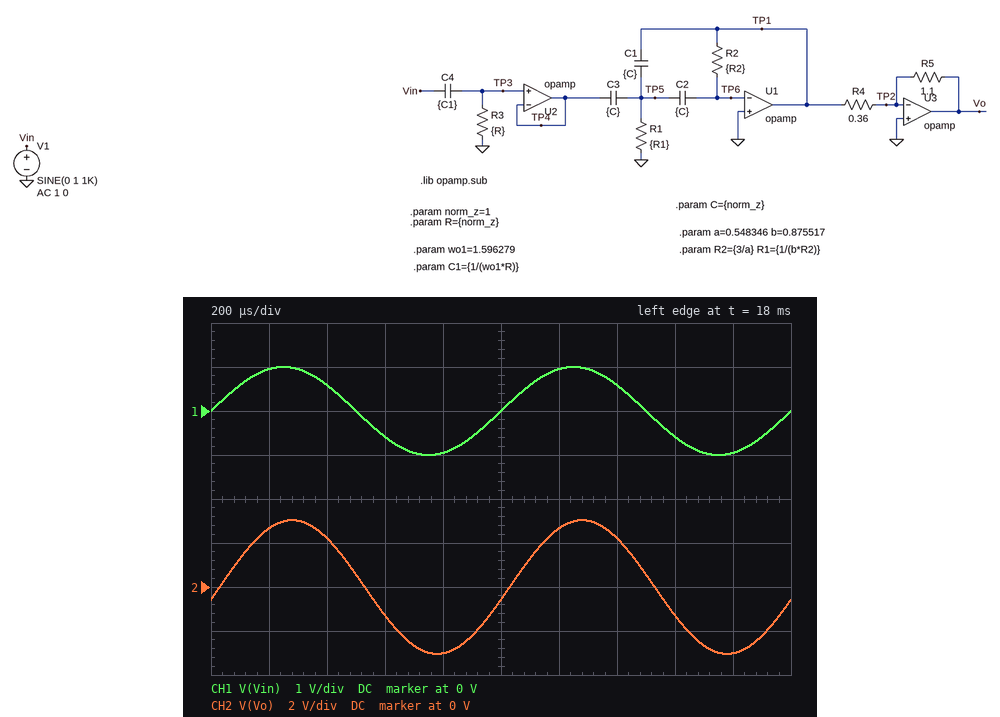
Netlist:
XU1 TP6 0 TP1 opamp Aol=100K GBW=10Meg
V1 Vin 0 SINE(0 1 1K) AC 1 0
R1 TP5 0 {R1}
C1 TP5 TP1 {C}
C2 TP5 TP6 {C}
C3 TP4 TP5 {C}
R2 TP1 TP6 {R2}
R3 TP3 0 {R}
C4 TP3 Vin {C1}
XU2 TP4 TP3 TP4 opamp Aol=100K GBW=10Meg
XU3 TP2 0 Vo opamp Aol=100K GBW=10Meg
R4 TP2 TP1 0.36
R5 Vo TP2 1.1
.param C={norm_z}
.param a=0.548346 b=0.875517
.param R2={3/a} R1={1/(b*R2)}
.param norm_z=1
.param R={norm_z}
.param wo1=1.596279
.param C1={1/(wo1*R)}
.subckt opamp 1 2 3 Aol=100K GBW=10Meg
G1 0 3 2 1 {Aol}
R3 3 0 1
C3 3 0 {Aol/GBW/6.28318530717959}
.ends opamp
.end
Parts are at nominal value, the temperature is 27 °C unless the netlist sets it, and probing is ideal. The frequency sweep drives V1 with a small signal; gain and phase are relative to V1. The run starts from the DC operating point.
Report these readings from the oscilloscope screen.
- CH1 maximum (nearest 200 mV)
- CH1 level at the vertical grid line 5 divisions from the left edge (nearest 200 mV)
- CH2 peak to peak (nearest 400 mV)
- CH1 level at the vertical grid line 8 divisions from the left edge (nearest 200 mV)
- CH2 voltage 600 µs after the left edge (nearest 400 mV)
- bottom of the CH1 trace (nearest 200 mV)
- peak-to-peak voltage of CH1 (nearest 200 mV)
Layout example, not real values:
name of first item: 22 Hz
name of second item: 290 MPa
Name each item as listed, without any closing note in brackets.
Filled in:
CH1 maximum: 1.0 V
CH1 level at the vertical grid line 5 divisions from the left edge: 0 V
CH2 peak to peak: 6.0 V
CH1 level at the vertical grid line 8 divisions from the left edge: -600 mV
CH2 voltage 600 µs after the left edge: -1.2 V
bottom of the CH1 trace: -1.0 V
peak-to-peak voltage of CH1: 2.0 V
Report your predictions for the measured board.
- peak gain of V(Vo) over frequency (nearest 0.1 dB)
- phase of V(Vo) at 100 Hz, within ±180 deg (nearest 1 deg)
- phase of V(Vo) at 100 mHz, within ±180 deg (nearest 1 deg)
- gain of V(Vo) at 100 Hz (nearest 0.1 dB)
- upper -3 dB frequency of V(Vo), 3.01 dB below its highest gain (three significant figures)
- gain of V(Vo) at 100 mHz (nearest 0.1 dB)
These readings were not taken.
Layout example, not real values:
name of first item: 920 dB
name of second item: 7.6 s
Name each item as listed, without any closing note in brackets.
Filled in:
peak gain of V(Vo) over frequency: 9.7 dB
phase of V(Vo) at 100 Hz, within ±180 deg: -1 deg
phase of V(Vo) at 100 mHz, within ±180 deg: -147 deg
gain of V(Vo) at 100 Hz: 9.7 dB
upper -3 dB frequency of V(Vo), 3.01 dB below its highest gain: 11.2 kHz
gain of V(Vo) at 100 mHz: -2.5 dB
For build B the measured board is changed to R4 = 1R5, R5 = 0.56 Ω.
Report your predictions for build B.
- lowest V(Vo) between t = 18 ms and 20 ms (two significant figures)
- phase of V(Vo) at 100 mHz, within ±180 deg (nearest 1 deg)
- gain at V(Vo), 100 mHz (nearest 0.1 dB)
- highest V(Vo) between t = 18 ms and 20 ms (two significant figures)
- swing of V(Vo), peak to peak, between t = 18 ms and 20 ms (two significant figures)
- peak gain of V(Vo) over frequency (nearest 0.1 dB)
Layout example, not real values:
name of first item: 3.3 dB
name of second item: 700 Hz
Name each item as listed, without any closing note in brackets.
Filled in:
lowest V(Vo) between t = 18 ms and 20 ms: -370 mV
phase of V(Vo) at 100 mHz, within ±180 deg: -147 deg
gain at V(Vo), 100 mHz: -20.8 dB
highest V(Vo) between t = 18 ms and 20 ms: 370 mV
swing of V(Vo), peak to peak, between t = 18 ms and 20 ms: 740 mV
peak gain of V(Vo) over frequency: -8.6 dB
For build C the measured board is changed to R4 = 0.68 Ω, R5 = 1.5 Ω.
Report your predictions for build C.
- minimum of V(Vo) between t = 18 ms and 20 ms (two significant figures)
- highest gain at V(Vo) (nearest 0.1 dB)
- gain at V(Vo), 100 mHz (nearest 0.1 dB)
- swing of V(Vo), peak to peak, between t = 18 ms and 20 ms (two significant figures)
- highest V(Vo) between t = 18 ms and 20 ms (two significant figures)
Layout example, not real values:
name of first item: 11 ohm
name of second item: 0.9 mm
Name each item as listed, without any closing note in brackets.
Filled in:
minimum of V(Vo) between t = 18 ms and 20 ms: -2.2 V
highest gain at V(Vo): 6.9 dB
gain at V(Vo), 100 mHz: -5.4 dB
swing of V(Vo), peak to peak, between t = 18 ms and 20 ms: 4.4 V
highest V(Vo) between t = 18 ms and 20 ms: 2.2 V
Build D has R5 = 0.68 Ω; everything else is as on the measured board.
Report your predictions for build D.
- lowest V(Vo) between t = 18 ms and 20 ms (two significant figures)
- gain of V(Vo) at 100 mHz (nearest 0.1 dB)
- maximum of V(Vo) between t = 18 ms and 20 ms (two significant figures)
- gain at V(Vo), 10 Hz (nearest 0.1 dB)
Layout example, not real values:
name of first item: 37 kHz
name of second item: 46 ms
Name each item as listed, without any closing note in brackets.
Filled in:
lowest V(Vo) between t = 18 ms and 20 ms: -1.9 V
gain of V(Vo) at 100 mHz: -6.7 dB
maximum of V(Vo) between t = 18 ms and 20 ms: 1.9 V
gain at V(Vo), 10 Hz: 5.5 dB
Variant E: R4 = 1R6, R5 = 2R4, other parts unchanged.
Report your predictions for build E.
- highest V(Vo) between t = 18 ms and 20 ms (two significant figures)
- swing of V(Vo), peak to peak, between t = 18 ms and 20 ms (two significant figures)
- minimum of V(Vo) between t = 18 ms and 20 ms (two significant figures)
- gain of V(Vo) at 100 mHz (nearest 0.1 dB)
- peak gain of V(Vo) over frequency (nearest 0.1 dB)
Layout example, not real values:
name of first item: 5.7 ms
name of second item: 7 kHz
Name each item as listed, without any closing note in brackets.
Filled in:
highest V(Vo) between t = 18 ms and 20 ms: 1.5 V
swing of V(Vo), peak to peak, between t = 18 ms and 20 ms: 3.0 V
minimum of V(Vo) between t = 18 ms and 20 ms: -1.5 V
gain of V(Vo) at 100 mHz: -8.7 dB
peak gain of V(Vo) over frequency: 3.5 dB
